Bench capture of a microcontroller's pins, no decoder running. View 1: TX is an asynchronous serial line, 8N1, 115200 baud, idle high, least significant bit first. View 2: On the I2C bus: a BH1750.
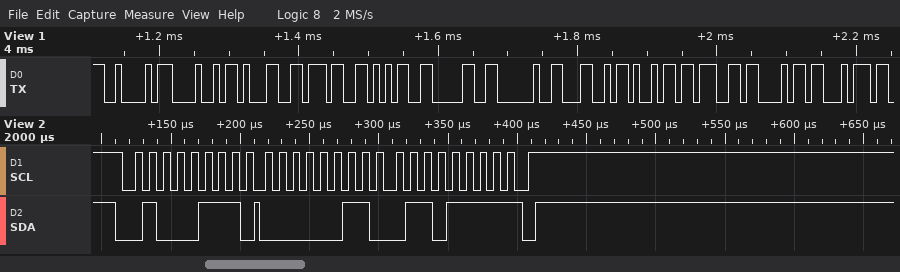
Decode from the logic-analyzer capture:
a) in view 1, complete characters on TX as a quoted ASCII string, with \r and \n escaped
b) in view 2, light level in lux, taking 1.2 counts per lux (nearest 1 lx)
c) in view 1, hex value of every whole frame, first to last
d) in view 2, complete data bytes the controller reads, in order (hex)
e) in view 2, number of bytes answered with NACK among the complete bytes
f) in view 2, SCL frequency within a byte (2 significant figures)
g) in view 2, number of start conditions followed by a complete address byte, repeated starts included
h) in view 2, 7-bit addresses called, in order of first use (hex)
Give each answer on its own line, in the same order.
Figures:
"BH1750 Light"
732 lx
42 48 31 37 35 30 20 4C 69 67 68 74
03 6F
1
100 kHz
1
0x23
